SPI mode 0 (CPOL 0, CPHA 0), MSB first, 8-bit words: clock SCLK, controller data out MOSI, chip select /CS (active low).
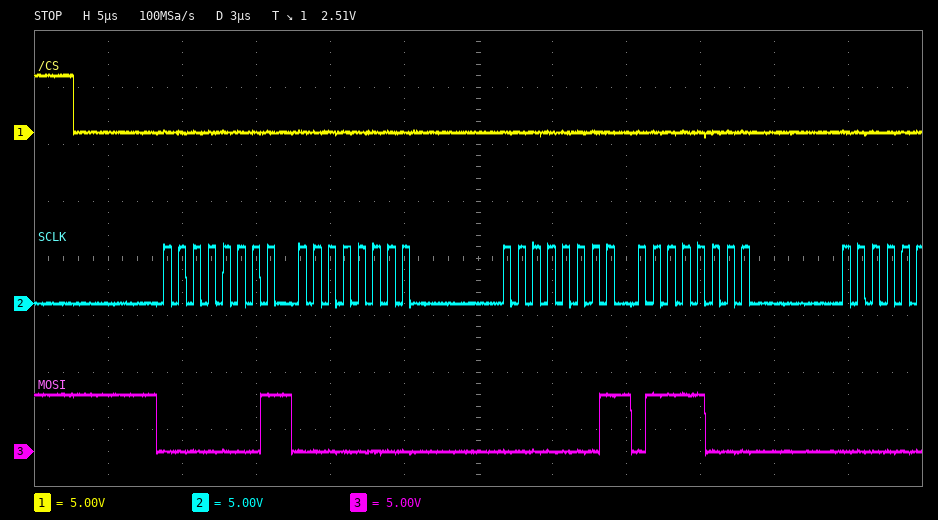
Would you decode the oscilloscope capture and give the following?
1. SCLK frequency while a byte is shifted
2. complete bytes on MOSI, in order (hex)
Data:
1 MHz
01 00 01 78
